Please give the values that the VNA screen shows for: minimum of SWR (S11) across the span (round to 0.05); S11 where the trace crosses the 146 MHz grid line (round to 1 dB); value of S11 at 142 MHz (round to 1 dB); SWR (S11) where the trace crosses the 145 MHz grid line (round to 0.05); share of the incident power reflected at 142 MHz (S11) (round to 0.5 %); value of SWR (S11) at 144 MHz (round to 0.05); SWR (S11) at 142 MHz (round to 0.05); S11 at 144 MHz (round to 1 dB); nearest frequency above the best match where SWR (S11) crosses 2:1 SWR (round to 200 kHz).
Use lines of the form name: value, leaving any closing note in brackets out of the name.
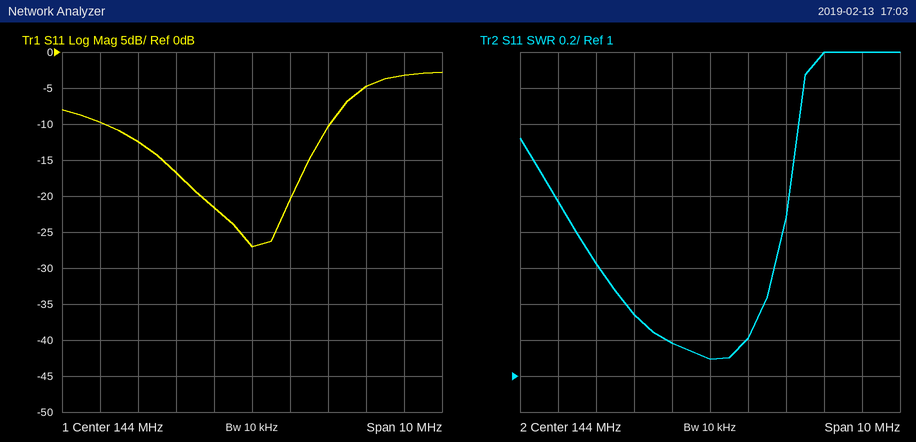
minimum of SWR (S11) across the span: 1.10
S11 where the trace crosses the 146 MHz grid line: -10 dB
value of S11 at 142 MHz: -17 dB
SWR (S11) where the trace crosses the 145 MHz grid line: 1.20
share of the incident power reflected at 142 MHz (S11): 2.0 %
value of SWR (S11) at 144 MHz: 1.10
SWR (S11) at 142 MHz: 1.35
S11 at 144 MHz: -27 dB
nearest frequency above the best match where SWR (S11) crosses 2:1 SWR: 146.0 MHz
